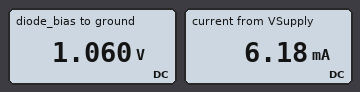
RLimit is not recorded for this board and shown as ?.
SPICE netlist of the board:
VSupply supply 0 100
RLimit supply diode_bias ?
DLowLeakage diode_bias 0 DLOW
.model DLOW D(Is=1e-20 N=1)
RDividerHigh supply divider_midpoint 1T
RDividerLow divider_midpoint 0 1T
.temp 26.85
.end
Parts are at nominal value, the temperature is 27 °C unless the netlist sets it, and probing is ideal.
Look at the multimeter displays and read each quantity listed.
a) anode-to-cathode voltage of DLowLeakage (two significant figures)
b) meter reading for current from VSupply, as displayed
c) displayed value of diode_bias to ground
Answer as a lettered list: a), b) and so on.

a) 1.1 V
b) 6.18 mA
c) 1.060 V
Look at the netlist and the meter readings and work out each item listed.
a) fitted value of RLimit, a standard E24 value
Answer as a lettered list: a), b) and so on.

a) 16 kΩ
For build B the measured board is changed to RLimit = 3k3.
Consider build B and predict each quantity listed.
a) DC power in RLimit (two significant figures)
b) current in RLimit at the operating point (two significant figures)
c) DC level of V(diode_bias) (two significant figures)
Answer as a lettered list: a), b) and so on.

a) 3.0 W
b) 30 mA
c) 1.1 V
